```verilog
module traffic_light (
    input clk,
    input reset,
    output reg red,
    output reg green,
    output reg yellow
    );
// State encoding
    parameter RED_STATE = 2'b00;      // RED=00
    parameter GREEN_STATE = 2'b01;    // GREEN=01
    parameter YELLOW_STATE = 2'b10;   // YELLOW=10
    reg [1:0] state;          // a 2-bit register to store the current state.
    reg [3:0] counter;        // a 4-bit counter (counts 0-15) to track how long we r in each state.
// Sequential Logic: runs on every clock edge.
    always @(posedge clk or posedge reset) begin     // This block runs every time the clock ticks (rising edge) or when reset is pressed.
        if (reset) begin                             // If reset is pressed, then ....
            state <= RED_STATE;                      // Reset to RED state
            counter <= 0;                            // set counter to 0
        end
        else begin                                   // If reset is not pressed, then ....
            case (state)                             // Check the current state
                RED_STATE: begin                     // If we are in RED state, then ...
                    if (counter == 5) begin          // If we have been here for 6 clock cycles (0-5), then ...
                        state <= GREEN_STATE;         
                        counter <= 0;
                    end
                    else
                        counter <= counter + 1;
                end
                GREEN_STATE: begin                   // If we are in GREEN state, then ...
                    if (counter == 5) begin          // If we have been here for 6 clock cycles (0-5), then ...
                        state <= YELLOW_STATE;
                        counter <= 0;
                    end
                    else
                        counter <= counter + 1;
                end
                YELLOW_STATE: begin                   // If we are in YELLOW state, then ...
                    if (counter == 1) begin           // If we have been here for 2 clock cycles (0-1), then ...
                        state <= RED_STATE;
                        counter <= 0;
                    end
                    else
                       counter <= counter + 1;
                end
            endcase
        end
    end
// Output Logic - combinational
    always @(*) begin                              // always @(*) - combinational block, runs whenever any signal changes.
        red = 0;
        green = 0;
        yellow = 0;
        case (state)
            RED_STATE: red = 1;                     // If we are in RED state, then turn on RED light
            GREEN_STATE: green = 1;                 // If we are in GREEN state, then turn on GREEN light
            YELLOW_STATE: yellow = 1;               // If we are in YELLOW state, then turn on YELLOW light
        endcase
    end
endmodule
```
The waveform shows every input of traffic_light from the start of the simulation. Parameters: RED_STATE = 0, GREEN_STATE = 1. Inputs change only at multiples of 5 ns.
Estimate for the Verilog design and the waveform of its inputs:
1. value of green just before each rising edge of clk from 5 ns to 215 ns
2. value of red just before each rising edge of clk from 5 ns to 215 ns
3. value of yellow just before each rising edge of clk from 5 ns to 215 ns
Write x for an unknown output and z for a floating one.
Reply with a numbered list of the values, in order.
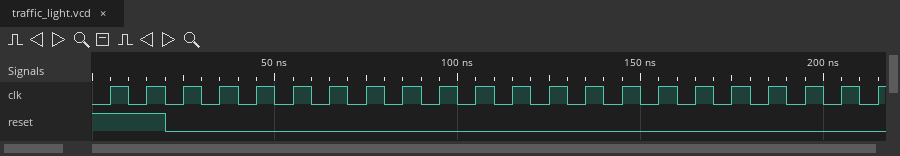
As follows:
1. 0 0 0 0 0 0 0 0 1 1 1 1 1 1 0 0 0 0 0 0 0 0
2. 1 1 1 1 1 1 1 1 0 0 0 0 0 0 0 0 1 1 1 1 1 1
3. 0 0 0 0 0 0 0 0 0 0 0 0 0 0 1 1 0 0 0 0 0 0
